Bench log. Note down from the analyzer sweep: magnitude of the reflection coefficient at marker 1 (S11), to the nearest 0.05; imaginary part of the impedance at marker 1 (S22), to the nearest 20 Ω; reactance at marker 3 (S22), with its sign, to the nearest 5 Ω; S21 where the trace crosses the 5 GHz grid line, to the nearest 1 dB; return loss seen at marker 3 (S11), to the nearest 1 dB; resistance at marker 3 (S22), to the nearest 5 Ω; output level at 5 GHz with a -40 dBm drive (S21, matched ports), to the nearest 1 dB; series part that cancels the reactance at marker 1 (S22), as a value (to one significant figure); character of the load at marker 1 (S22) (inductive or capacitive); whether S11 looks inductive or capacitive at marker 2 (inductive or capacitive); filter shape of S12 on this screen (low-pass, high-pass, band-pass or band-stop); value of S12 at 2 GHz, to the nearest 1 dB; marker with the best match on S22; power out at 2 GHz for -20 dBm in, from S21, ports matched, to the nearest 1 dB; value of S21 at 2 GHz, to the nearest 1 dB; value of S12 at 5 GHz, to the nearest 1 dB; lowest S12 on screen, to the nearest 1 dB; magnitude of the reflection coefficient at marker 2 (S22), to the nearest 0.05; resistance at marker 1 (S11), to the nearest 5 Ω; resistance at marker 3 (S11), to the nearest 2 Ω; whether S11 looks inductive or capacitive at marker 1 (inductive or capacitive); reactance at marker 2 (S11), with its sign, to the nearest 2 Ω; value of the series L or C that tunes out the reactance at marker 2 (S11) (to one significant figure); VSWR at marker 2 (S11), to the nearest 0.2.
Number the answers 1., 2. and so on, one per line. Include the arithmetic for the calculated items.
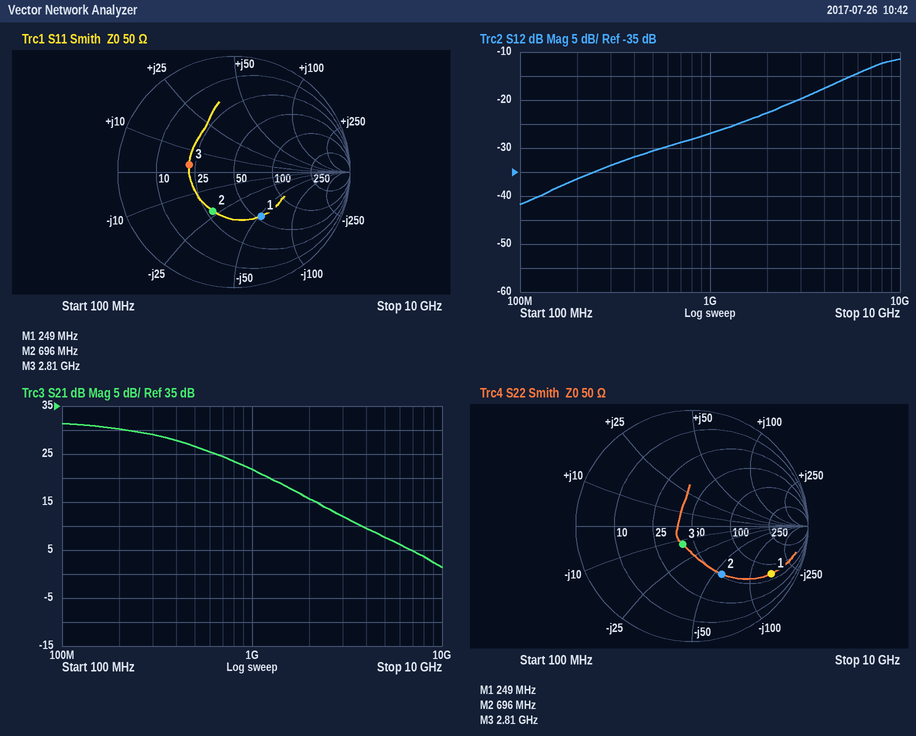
1. 0.45
2. -160 Ω
3. -15 Ω
4. 8 dB
5. 8 dB
6. 40 Ω
7. -40 dBm + (8 dB) = -32 dBm
8. L = 160 Ω/(2π × 249 MHz) ≈ 102 nH, so 100 nH to one significant figure
9. capacitive
10. capacitive
11. high-pass
12. -23 dB
13. marker 3
14. -20 dBm + (16 dB) = -4 dBm
15. 16 dB
16. -16 dB
17. -42 dB
18. 0.50
19. 55 Ω
20. 22 Ω
21. capacitive
22. -22 Ω
23. L = 22 Ω/(2π × 696 MHz) ≈ 5 nH
24. 2.2
